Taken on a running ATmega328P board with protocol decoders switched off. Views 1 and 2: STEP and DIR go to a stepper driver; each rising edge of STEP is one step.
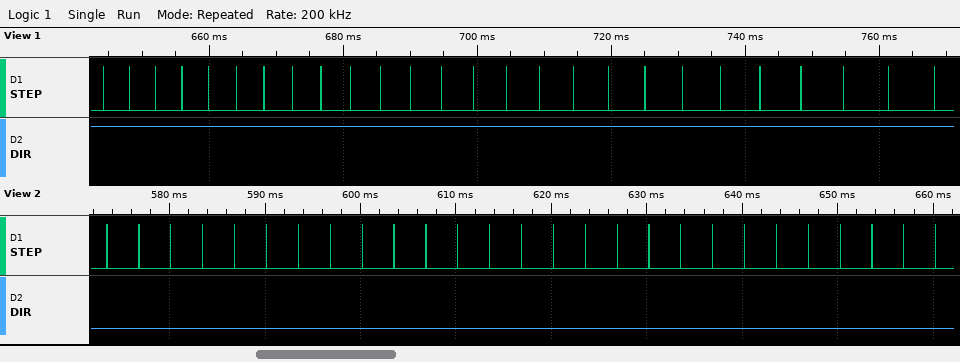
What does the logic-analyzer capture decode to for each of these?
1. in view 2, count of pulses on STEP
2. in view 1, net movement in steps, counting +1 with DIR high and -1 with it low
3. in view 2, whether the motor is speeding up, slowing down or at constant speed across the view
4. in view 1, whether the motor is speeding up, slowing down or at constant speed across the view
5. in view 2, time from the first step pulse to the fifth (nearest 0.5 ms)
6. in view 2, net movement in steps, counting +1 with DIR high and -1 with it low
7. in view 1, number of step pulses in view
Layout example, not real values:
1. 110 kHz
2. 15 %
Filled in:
1. 27
2. +26
3. constant speed
4. slowing down
5. 13.5 ms
6. -27
7. 26
